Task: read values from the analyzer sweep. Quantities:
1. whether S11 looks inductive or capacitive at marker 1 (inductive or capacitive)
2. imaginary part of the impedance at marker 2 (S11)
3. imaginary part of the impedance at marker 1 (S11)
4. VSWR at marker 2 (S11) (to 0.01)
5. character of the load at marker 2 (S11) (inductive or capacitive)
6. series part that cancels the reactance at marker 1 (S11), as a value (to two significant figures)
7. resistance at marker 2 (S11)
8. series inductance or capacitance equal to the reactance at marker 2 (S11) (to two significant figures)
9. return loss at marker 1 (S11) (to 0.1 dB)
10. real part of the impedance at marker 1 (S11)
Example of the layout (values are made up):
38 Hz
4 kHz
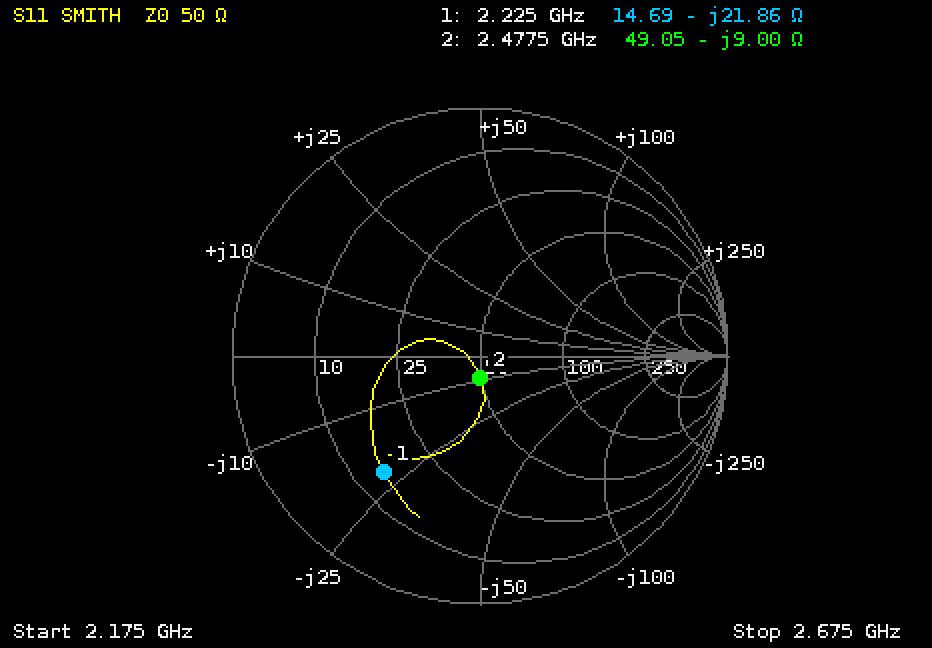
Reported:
capacitive
-9.00 Ω
-21.86 Ω
1.20
capacitive
1.6 nH
49.05 Ω
7.1 pF
4.3 dB
14.69 Ω
